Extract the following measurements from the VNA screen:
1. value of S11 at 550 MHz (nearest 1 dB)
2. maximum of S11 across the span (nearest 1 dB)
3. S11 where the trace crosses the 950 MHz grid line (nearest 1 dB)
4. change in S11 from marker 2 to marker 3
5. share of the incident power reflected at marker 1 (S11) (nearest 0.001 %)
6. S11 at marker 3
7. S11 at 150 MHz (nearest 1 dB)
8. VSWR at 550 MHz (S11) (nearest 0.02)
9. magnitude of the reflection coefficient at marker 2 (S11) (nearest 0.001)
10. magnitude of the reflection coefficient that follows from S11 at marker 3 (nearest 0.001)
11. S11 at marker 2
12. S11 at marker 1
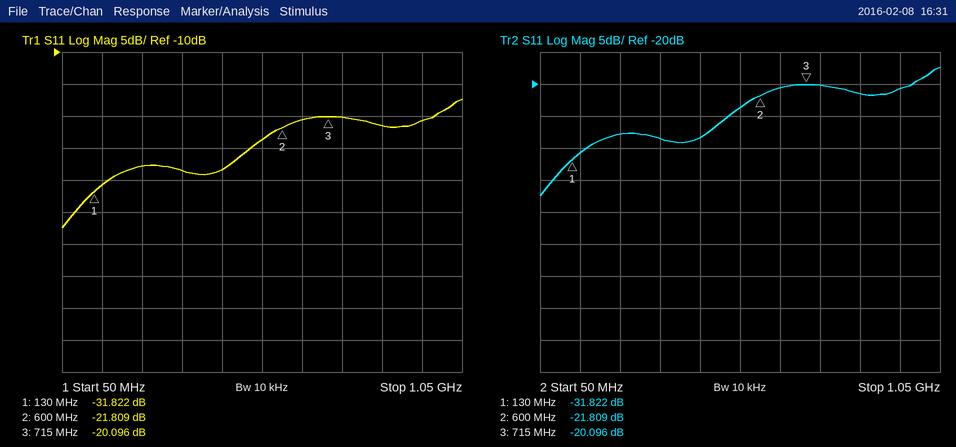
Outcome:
-24 dB
-17 dB
-21 dB
1.713 dB
0.066 %
-20.096 dB
-31 dB
1.14
0.081
0.099
-21.809 dB
-31.822 dB
